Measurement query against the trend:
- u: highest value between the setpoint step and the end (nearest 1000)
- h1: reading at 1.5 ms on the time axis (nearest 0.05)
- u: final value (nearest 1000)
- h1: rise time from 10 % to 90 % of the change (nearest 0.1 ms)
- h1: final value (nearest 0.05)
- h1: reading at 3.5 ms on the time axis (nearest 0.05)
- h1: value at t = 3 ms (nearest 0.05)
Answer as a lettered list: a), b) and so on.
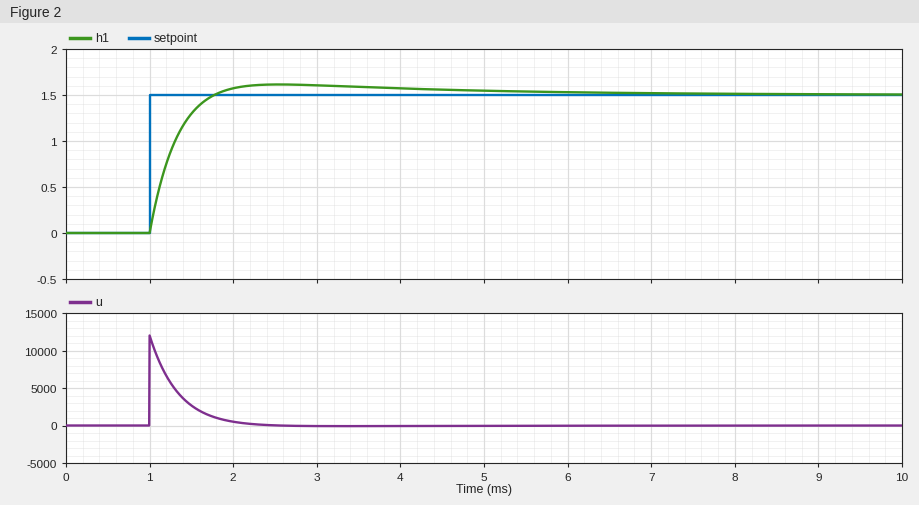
a) 12000
b) 1.30
c) 0
d) 0.5 ms
e) 1.50
f) 1.60
g) 1.60
